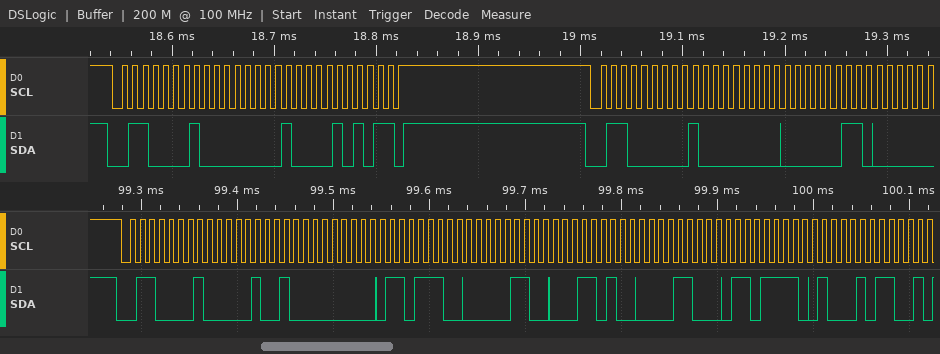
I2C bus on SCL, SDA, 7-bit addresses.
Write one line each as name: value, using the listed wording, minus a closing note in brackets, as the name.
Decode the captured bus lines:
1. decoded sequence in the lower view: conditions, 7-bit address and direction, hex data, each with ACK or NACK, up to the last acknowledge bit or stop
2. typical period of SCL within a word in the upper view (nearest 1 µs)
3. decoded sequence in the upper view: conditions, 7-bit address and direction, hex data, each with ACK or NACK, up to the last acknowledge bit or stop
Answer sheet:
decoded sequence in the lower view: conditions, 7-bit address and direction, hex data, each with ACK or NACK, up to the last acknowledge bit or stop: start, address 30 read ACK, 09 ACK, 00 ACK, DC ACK, 0C ACK, 34 ACK, 18 ACK, DE ACK, 8B ACK
typical period of SCL within a word in the upper view: 10 µs
decoded sequence in the upper view: conditions, 7-bit address and direction, hex data, each with ACK or NACK, up to the last acknowledge bit or stop: start, address 30 read ACK, 01 ACK, 15 NACK, stop, start, address 30 write ACK, 80 ACK, 03 ACK
